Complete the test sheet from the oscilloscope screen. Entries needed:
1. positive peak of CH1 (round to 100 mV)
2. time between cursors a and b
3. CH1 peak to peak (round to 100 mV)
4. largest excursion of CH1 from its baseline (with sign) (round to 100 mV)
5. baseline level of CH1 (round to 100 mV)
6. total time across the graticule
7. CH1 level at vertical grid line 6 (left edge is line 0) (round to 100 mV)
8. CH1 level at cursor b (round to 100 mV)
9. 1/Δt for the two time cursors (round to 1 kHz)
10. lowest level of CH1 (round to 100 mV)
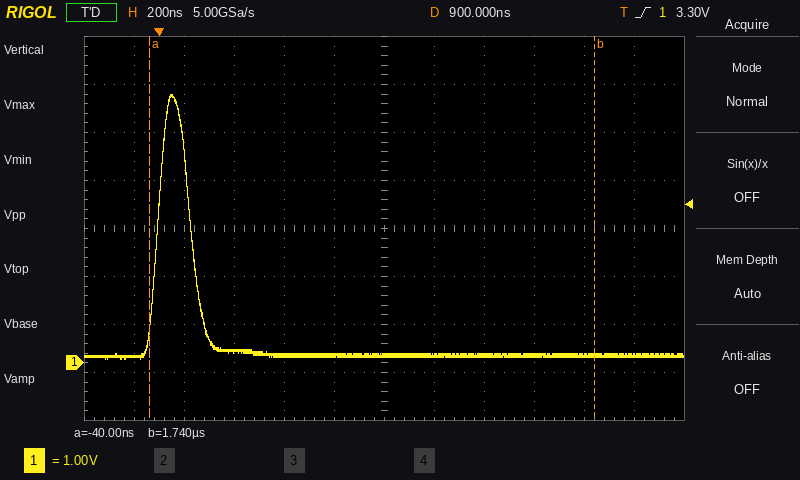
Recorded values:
5.6 V
1.78 µs
5.5 V
+5.4 V
200 mV
2.4 µs
200 mV
200 mV
562 kHz
100 mV
